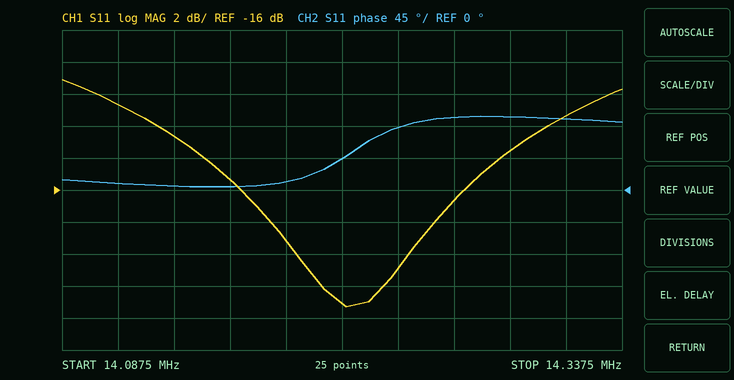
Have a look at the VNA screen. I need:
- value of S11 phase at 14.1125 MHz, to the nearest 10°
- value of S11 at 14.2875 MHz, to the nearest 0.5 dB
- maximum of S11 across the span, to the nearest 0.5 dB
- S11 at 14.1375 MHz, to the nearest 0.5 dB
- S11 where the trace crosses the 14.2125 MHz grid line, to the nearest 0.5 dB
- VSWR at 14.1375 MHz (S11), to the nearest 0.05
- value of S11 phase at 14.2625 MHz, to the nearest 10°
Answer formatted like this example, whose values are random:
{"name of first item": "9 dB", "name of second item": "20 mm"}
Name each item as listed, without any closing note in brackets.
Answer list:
{"value of S11 phase at 14.1125 MHz, to the nearest 10°": "10°", "value of S11 at 14.2875 MHz, to the nearest 0.5 dB": "-13.5 dB", "maximum of S11 across the span, to the nearest 0.5 dB": "-9.0 dB", "S11 at 14.1375 MHz, to the nearest 0.5 dB": "-12.5 dB", "S11 where the trace crosses the 14.2125 MHz grid line, to the nearest 0.5 dB": "-23.0 dB", "VSWR at 14.1375 MHz (S11), to the nearest 0.05": "1.60", "value of S11 phase at 14.2625 MHz, to the nearest 10°": "100°"}
